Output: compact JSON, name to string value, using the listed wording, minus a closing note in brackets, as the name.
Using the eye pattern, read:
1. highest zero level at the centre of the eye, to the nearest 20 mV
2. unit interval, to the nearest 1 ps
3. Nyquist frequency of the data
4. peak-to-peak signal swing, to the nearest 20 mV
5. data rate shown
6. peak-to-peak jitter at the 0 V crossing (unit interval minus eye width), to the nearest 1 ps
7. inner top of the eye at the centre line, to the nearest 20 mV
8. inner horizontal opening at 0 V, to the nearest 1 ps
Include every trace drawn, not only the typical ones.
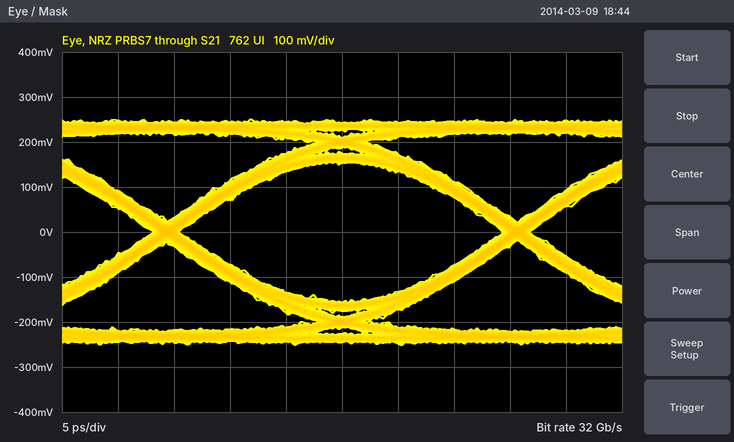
{"highest zero level at the centre of the eye, to the nearest 20 mV": "-160 mV", "unit interval, to the nearest 1 ps": "31 ps", "Nyquist frequency of the data": "16 GHz", "peak-to-peak signal swing, to the nearest 20 mV": "500 mV", "data rate shown": "32 Gb/s", "peak-to-peak jitter at the 0 V crossing (unit interval minus eye width), to the nearest 1 ps": "2 ps", "inner top of the eye at the centre line, to the nearest 20 mV": "160 mV", "inner horizontal opening at 0 V, to the nearest 1 ps": "29 ps"}
